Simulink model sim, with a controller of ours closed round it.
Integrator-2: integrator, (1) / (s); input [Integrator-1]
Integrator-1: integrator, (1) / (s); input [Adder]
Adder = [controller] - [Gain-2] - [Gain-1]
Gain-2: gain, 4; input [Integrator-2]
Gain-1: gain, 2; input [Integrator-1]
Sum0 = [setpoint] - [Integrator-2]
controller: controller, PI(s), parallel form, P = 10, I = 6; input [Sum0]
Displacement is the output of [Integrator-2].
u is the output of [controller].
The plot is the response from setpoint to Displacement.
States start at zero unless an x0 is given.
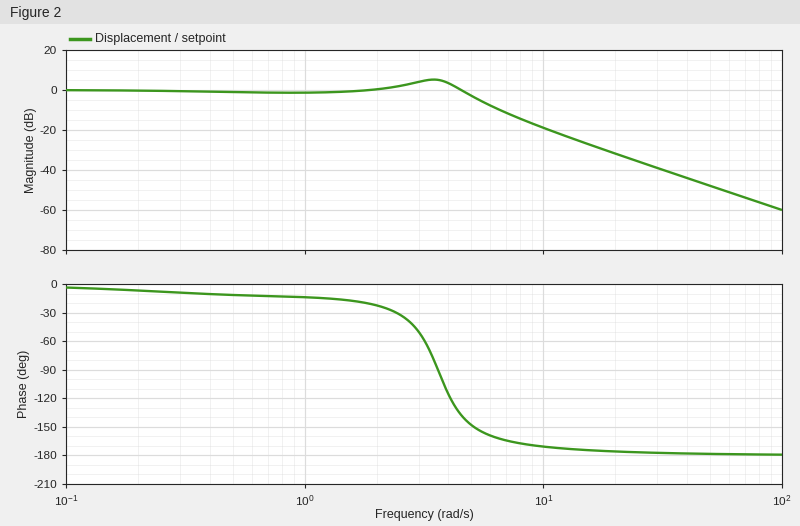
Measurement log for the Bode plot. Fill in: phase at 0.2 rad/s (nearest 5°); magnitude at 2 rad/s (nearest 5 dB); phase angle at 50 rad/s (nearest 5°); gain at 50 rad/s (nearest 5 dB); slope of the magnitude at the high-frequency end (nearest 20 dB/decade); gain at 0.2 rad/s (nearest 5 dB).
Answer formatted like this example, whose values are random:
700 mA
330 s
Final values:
-5°
0 dB
-180°
-50 dB
-40 dB/decade
0 dB
